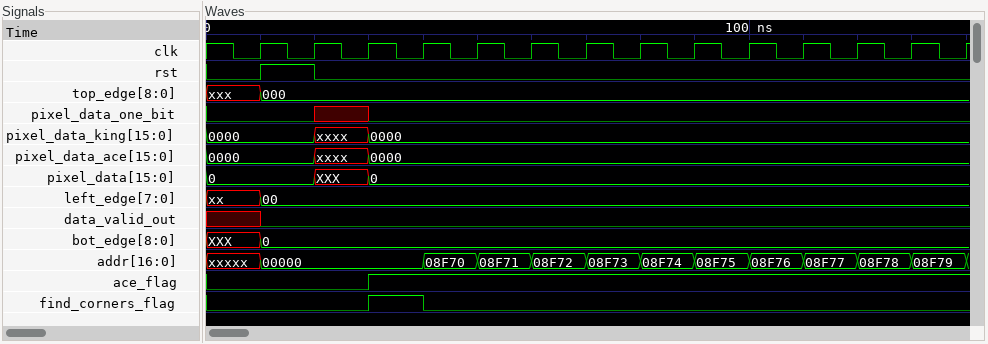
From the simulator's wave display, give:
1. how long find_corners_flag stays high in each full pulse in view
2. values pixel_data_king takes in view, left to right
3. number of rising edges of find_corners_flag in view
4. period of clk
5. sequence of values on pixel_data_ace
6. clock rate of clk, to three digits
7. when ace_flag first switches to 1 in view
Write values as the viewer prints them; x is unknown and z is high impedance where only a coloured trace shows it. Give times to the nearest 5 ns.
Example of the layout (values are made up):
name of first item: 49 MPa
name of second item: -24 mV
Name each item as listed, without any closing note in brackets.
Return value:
how long find_corners_flag stays high in each full pulse in view: 10 ns
values pixel_data_king takes in view, left to right: 0000, xxxx, 0000
number of rising edges of find_corners_flag in view: 1
period of clk: 10 ns
sequence of values on pixel_data_ace: 0000, xxxx, 0000
clock rate of clk, to three digits: 100 MHz
when ace_flag first switches to 1 in view: 30 ns
